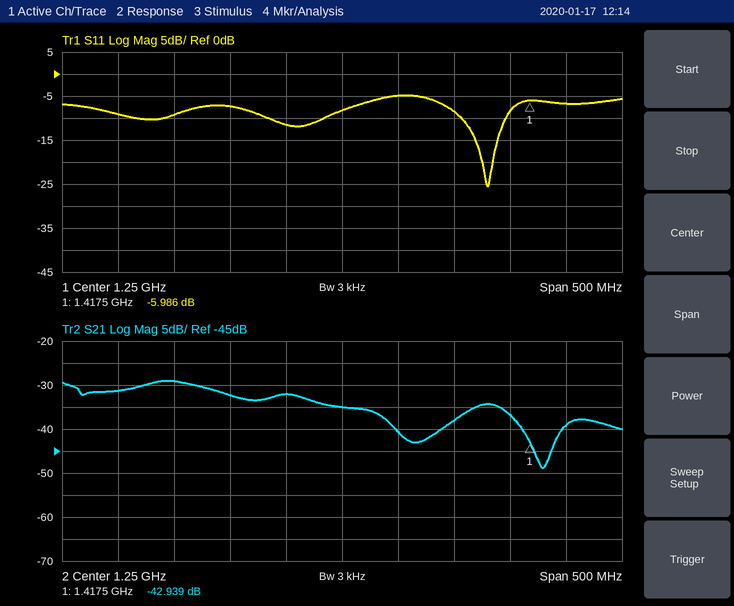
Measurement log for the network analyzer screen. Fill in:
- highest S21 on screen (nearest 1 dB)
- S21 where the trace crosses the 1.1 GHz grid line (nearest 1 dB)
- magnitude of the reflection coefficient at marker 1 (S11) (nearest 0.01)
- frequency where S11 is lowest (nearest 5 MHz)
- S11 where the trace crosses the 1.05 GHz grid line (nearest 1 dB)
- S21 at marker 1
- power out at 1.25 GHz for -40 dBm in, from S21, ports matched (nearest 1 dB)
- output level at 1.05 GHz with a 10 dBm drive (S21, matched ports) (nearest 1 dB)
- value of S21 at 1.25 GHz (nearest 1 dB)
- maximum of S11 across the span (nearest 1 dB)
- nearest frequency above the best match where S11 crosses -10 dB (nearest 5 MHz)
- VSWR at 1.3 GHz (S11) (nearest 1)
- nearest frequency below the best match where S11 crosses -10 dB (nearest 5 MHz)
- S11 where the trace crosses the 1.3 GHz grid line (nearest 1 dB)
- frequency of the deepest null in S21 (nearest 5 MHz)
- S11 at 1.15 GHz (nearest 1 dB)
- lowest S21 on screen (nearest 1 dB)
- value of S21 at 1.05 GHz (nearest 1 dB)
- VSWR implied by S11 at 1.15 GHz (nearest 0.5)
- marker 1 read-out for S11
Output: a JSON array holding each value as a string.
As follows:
["-29 dB", "-29 dB", "0.50", "1.380 GHz", "-9 dB", "-42.939 dB", "-75 dBm", "-21 dBm", "-35 dB", "-5 dB", "1.395 GHz", "4", "1.355 GHz", "-5 dB", "1.430 GHz", "-7 dB", "-49 dB", "-31 dB", "2.5", "-5.986 dB"]
